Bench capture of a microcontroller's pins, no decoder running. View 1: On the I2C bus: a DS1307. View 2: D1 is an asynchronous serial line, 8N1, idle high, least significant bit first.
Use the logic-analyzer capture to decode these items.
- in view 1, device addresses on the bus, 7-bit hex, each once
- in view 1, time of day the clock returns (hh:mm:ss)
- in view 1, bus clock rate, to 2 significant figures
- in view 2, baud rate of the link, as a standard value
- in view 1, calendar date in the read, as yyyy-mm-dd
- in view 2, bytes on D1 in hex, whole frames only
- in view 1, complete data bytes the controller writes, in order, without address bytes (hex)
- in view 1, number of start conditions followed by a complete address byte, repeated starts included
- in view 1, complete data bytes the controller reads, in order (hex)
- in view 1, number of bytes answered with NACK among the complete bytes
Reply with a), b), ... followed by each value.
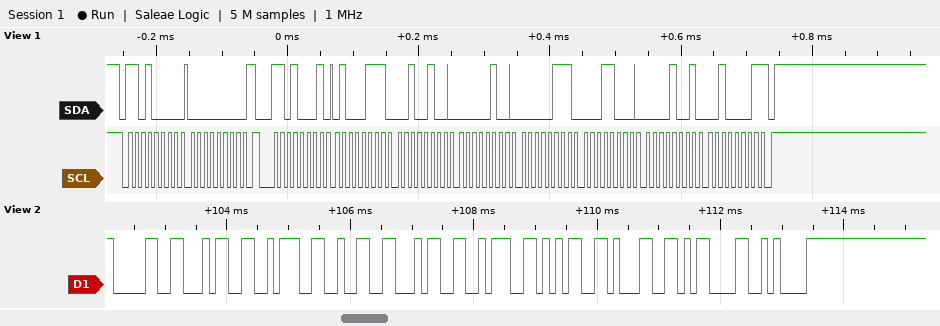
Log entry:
a) 0x68
b) 04:24:47
c) 100 kHz
d) 9600 baud
e) 2021-09-18
f) 0x30 0x34 0x3A 0x32 0x34 0x3A 0x35 0x31 0x0D 0x0A
g) 00
h) 2
i) 47 24 04 07 18 09 21
j) 1
